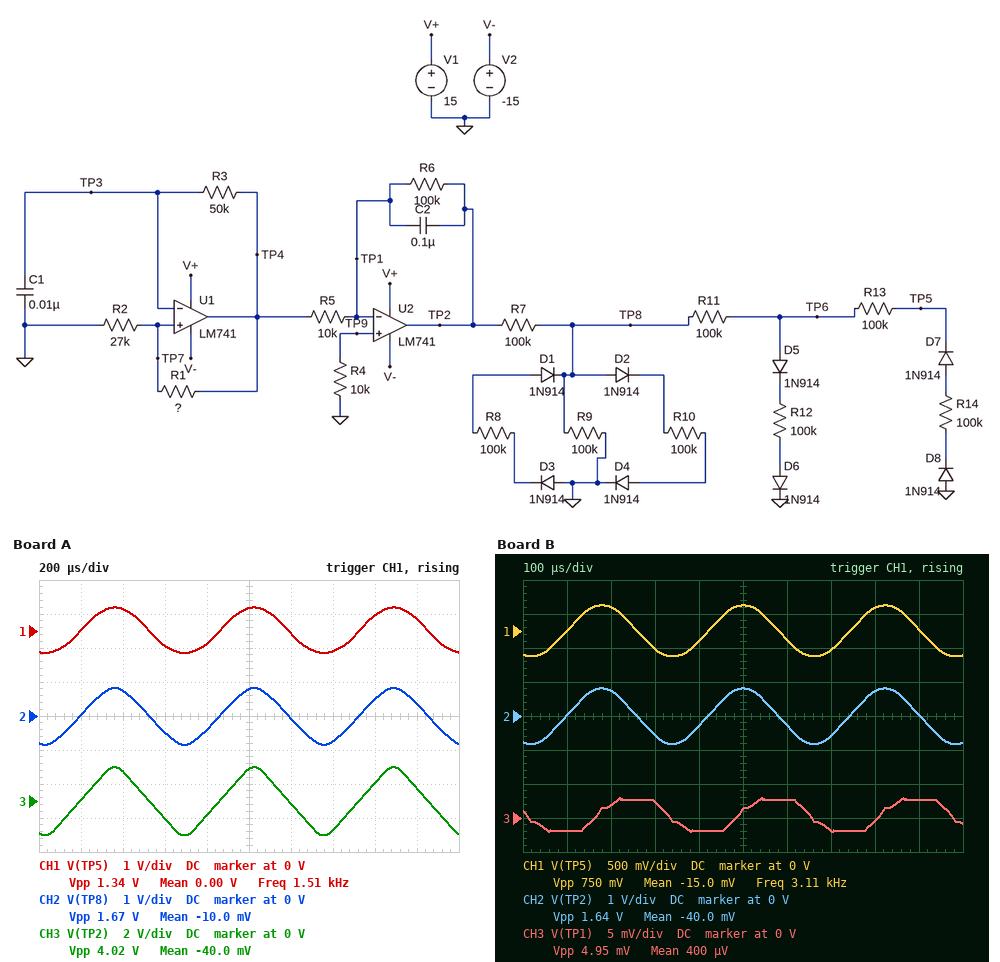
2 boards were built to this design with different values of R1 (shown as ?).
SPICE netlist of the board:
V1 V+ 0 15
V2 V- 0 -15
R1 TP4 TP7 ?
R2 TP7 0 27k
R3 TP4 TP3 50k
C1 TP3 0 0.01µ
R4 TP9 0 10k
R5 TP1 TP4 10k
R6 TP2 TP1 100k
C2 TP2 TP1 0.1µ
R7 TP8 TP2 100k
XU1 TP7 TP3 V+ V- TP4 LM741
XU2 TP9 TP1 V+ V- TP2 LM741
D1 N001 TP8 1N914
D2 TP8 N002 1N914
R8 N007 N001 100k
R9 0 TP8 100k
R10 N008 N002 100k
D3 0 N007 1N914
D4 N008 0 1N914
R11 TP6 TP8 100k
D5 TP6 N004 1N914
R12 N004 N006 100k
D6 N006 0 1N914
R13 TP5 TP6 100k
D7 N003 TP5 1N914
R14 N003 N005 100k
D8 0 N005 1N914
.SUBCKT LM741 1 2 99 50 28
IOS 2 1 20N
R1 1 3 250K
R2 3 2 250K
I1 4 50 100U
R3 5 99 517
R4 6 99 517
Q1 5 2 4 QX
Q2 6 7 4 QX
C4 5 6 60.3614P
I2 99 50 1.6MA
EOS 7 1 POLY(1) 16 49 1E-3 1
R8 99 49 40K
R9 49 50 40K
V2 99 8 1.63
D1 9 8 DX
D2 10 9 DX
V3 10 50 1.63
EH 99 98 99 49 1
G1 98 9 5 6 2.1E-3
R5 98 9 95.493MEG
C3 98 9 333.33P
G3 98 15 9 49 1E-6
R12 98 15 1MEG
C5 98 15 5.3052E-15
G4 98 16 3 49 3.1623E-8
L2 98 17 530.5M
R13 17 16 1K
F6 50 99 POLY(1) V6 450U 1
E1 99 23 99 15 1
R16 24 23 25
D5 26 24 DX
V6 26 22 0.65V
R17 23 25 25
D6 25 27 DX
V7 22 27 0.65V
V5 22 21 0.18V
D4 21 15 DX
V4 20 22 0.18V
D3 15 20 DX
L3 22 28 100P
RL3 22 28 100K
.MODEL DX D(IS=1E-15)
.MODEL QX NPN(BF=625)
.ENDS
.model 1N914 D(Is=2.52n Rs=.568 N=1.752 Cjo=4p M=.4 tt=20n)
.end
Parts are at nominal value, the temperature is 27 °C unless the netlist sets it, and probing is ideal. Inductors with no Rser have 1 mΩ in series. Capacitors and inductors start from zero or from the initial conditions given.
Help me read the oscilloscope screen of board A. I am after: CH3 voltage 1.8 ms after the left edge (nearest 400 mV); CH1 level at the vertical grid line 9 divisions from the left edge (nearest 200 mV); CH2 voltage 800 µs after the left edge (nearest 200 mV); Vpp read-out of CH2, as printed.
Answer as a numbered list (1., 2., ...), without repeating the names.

1. 800 mV
2. 400 mV
3. -400 mV
4. 1.67 V
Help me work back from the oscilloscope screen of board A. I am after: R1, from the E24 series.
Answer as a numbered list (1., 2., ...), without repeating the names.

1. 75 kΩ
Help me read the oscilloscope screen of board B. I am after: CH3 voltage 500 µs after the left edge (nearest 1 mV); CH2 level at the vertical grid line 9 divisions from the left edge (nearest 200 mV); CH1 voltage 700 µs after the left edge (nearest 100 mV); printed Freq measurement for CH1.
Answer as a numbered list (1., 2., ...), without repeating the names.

1. 1 mV
2. 0 V
3. -300 mV
4. 3.11 kHz
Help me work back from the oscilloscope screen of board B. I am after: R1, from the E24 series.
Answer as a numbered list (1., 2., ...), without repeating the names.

1. 300 kΩ
